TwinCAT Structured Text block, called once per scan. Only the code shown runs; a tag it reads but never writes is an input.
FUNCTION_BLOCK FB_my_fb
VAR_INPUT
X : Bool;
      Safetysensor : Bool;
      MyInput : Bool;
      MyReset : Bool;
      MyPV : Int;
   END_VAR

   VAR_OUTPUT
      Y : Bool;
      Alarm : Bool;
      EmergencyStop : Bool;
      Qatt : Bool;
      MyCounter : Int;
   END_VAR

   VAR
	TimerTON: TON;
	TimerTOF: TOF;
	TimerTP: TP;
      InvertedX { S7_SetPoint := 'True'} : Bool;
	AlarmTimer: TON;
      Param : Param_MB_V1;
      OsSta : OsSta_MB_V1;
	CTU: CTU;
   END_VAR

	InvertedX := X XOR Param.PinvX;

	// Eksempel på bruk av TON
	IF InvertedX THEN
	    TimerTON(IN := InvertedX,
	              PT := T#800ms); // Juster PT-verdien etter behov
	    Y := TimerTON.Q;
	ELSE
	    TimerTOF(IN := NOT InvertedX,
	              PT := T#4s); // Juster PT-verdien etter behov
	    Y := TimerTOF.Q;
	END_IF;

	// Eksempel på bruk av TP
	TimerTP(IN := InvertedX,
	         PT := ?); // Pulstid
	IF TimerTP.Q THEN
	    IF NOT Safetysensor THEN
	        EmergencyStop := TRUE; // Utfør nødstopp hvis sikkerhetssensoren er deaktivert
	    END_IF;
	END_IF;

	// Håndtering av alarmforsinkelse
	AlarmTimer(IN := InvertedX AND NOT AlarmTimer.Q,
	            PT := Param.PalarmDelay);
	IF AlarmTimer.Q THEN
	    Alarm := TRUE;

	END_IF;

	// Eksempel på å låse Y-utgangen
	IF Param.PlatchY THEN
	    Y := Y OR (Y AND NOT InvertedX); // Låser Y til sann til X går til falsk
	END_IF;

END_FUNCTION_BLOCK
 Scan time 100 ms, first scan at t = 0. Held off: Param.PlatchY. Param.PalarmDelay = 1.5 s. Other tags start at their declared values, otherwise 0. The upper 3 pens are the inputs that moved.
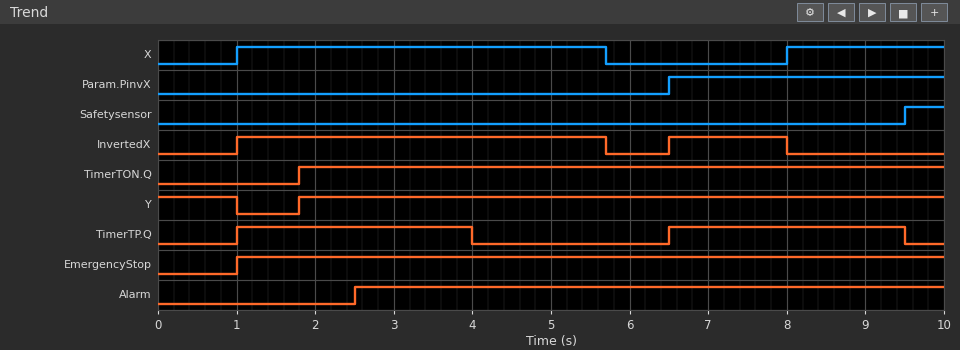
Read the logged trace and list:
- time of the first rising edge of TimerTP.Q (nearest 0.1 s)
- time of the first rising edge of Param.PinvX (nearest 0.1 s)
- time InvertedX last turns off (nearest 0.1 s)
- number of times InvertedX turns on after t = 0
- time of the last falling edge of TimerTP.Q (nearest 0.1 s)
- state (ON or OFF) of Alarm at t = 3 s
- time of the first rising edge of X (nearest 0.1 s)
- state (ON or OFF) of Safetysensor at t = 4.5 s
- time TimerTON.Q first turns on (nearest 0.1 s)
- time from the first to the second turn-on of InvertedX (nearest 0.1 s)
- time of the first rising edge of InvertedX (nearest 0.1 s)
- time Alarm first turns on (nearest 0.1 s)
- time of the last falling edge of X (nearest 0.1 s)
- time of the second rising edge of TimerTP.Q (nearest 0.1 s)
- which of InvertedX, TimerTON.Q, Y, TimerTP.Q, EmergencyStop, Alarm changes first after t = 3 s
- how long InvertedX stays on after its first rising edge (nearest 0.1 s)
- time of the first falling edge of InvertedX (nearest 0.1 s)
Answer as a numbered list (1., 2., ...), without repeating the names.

1. 1.0 s
2. 6.5 s
3. 8.0 s
4. 2
5. 9.5 s
6. ON
7. 1.0 s
8. OFF
9. 1.8 s
10. 5.5 s
11. 1.0 s
12. 2.5 s
13. 5.7 s
14. 6.5 s
15. TimerTP.Q
16. 4.7 s
17. 5.7 s
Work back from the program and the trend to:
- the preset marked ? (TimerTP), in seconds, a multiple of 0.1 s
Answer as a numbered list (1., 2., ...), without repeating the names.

1. 3.0 s
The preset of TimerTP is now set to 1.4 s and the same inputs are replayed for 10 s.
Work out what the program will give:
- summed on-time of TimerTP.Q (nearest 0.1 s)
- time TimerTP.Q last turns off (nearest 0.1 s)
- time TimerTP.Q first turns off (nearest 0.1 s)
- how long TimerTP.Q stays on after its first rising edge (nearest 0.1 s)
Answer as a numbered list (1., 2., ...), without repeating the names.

1. 2.8 s
2. 7.9 s
3. 2.4 s
4. 1.4 s
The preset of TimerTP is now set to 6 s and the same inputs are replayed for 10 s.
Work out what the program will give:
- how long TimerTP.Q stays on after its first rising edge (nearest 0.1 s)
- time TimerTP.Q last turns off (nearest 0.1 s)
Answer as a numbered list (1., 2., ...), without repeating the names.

1. 6.0 s
2. 7.0 s
